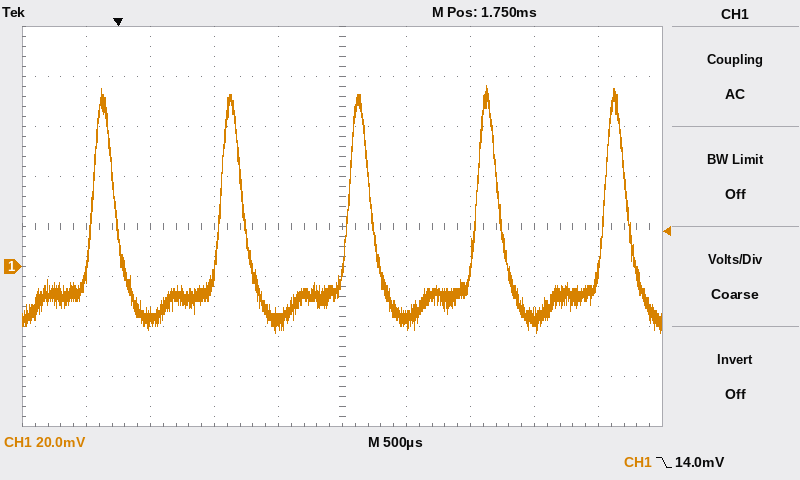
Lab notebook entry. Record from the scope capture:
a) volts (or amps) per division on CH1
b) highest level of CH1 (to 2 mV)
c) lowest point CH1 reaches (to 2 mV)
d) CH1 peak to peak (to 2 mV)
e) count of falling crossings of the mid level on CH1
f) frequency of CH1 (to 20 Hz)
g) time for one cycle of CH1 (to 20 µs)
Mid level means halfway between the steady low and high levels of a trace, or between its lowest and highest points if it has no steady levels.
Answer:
20 mV
72 mV
-26 mV
98 mV
5
1.00 kHz
1.00 ms
